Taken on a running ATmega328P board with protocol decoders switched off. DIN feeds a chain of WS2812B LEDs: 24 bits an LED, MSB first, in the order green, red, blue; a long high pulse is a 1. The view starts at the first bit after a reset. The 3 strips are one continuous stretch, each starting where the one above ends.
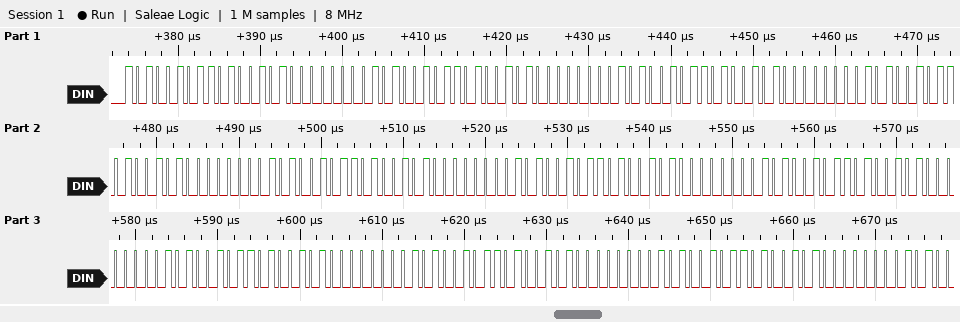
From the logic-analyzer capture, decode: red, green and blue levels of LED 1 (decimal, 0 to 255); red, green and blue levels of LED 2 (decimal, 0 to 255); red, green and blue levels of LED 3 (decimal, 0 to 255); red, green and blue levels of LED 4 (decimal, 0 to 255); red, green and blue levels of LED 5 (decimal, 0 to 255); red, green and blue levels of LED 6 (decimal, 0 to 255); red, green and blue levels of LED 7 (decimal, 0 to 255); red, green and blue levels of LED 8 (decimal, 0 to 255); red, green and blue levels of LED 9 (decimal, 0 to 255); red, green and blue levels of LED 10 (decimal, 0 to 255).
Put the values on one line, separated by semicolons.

165, 165, 0; 165, 165, 0; 165, 165, 0; 165, 165, 0; 165, 165, 0; 165, 165, 0; 165, 165, 0; 165, 165, 0; 165, 165, 0; 165, 165, 0
